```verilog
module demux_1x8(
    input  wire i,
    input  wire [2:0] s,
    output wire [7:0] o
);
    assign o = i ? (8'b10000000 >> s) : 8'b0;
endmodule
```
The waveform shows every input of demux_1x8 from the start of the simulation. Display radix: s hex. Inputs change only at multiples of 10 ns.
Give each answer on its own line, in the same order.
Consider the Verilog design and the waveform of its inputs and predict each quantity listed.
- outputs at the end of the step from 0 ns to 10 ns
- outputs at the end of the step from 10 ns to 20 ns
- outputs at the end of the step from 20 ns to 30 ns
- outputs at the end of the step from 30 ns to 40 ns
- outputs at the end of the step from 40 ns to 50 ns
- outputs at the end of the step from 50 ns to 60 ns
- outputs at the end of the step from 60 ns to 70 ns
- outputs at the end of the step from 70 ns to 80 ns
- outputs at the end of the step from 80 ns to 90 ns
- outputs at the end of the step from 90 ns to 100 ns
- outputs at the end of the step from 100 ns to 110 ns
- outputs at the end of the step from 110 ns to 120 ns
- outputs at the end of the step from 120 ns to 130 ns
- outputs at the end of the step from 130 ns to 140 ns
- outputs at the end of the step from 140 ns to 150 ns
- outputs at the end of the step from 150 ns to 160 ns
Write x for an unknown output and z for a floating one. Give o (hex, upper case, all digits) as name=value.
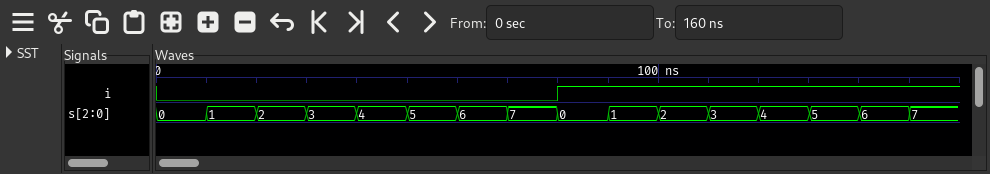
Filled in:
o=00
o=00
o=00
o=00
o=00
o=00
o=00
o=00
o=80
o=40
o=20
o=10
o=08
o=04
o=02
o=01
